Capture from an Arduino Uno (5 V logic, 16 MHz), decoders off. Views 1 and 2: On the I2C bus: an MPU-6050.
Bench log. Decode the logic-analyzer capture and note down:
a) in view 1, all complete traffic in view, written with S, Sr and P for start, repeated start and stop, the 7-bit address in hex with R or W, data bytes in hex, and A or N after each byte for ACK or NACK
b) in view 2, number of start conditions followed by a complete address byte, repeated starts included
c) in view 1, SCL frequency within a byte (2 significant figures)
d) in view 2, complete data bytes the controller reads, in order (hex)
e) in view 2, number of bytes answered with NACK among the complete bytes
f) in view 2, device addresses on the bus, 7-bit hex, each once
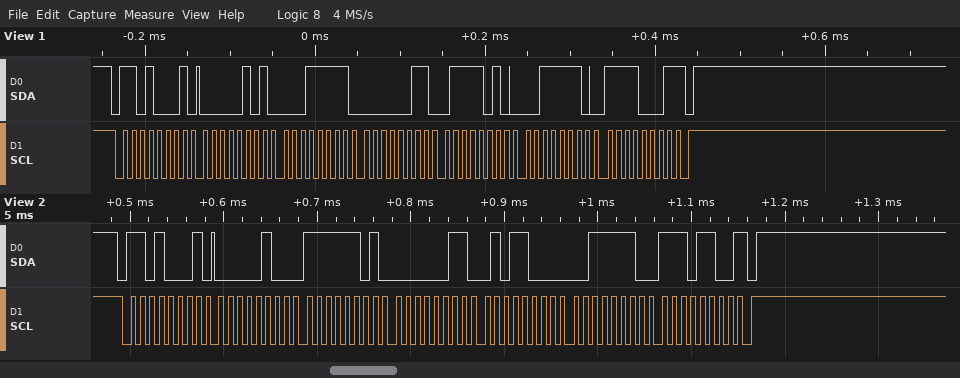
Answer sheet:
S 68R A 05 A 1F A 03 A 7A A 3E A F1 N P
1
100 kHz
04 FD 03 58 3E EC
1
0x68
